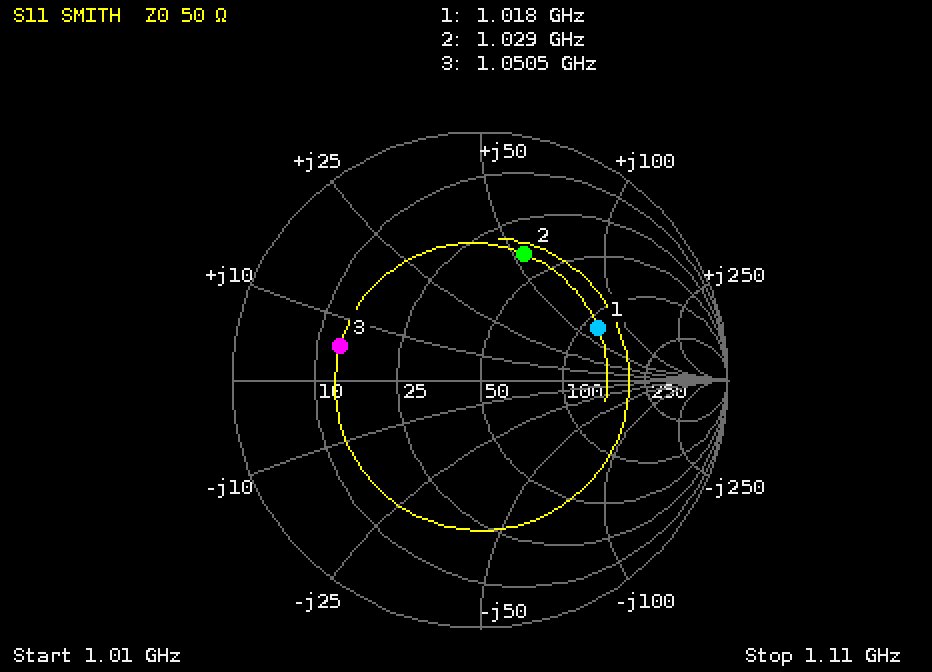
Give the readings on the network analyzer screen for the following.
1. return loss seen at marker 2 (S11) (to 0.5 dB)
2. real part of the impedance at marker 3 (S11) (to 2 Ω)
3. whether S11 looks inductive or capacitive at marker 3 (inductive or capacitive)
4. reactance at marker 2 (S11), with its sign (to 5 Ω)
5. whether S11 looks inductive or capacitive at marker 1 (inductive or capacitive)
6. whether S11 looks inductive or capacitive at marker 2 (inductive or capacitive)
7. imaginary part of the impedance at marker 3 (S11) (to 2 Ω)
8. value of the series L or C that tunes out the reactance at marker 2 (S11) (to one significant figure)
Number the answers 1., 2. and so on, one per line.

1. 5.5 dB
2. 14 Ω
3. inductive
4. +55 Ω
5. inductive
6. inductive
7. +6 Ω
8. 3 pF
